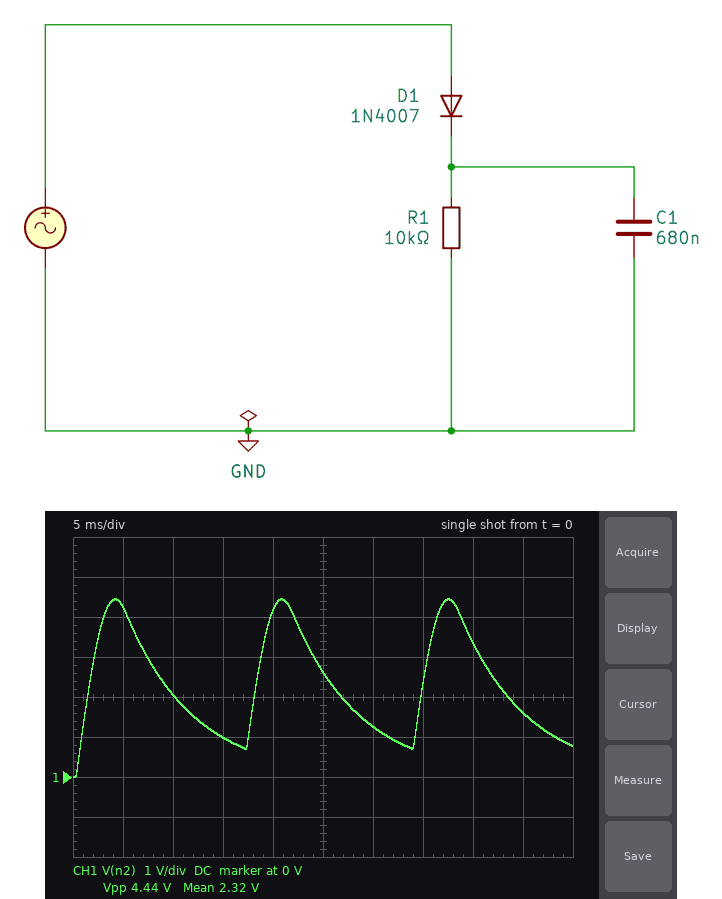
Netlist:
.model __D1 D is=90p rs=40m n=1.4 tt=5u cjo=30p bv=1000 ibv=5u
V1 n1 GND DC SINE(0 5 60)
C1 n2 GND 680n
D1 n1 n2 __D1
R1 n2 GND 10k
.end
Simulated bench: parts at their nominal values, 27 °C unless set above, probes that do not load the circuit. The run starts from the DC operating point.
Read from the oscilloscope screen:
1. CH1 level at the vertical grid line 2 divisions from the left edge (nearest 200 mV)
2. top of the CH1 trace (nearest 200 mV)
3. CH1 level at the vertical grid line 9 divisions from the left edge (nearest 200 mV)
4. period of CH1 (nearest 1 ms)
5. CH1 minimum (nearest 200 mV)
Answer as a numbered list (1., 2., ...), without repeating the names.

1. 2.0 V
2. 4.4 V
3. 1.6 V
4. 17 ms
5. 0 V
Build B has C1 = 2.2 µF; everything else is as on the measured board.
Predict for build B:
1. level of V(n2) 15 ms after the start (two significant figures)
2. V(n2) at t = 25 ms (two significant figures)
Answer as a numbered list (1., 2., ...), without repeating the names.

1. 2.8 V
2. 3.7 V
